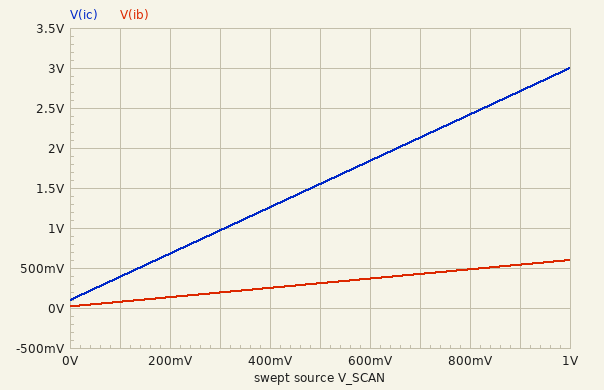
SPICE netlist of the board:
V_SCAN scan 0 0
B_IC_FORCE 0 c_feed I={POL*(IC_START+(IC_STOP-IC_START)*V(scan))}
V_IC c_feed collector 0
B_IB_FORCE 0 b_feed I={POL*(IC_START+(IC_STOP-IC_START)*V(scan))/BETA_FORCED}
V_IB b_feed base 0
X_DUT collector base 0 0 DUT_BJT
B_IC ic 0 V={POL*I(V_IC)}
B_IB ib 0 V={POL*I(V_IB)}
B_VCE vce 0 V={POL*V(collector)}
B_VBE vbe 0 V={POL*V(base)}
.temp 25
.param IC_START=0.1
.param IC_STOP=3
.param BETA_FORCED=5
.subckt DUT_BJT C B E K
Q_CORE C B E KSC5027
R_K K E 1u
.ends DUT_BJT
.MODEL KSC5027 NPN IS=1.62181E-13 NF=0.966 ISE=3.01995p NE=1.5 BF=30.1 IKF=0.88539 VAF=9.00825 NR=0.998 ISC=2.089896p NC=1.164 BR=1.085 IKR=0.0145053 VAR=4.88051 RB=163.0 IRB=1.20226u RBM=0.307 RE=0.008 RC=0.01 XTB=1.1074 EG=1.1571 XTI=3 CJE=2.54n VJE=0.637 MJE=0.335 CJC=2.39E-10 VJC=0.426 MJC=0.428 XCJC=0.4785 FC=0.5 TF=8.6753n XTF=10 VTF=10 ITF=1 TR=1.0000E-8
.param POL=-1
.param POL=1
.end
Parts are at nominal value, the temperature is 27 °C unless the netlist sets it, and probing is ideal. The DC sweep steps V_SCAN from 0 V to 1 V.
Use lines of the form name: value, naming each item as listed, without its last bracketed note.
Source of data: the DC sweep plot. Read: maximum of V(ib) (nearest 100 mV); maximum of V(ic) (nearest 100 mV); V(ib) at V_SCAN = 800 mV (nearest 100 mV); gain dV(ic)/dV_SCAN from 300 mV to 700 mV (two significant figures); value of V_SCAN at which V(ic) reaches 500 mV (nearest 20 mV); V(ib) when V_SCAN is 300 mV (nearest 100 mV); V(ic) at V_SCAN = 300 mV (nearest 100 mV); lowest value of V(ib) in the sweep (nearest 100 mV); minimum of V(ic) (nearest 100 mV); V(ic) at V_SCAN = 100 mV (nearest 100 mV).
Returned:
maximum of V(ib): 600 mV
maximum of V(ic): 3.0 V
V(ib) at V_SCAN = 800 mV: 500 mV
gain dV(ic)/dV_SCAN from 300 mV to 700 mV: 2.9 V/V
value of V_SCAN at which V(ic) reaches 500 mV: 140 mV
V(ib) when V_SCAN is 300 mV: 200 mV
V(ic) at V_SCAN = 300 mV: 1.0 V
lowest value of V(ib) in the sweep: 0 V
minimum of V(ic): 100 mV
V(ic) at V_SCAN = 100 mV: 400 mV
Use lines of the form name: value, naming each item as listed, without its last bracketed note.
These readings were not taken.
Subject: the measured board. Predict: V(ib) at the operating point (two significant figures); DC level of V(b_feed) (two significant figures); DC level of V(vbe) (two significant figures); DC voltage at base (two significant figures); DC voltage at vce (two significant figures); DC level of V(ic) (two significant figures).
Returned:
V(ib) at the operating point: 20 mV
DC level of V(b_feed): 730 mV
DC level of V(vbe): 730 mV
DC voltage at base: 730 mV
DC voltage at vce: 62 mV
DC level of V(ic): 100 mV
